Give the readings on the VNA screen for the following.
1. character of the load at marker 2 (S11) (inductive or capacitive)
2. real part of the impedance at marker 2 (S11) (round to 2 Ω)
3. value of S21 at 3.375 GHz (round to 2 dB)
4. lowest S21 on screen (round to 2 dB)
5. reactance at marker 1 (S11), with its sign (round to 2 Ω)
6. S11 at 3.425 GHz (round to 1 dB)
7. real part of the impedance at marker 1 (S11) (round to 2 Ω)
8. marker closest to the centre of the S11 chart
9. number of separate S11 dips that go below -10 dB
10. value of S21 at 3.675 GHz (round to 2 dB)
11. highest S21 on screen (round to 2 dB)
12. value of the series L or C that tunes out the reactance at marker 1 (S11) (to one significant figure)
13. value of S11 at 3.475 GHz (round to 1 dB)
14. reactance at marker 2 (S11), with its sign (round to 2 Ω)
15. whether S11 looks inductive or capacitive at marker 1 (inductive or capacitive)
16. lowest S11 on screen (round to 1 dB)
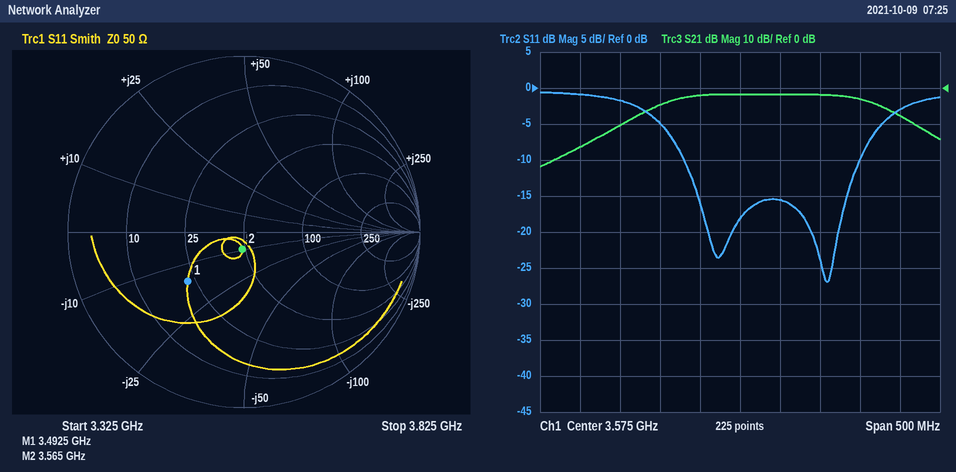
capacitive
48 Ω
-16 dB
-22 dB
-16 Ω
-2 dB
22 Ω
marker 2
2
-2 dB
-2 dB
700 pH
-5 dB
-10 Ω
capacitive
-27 dB
